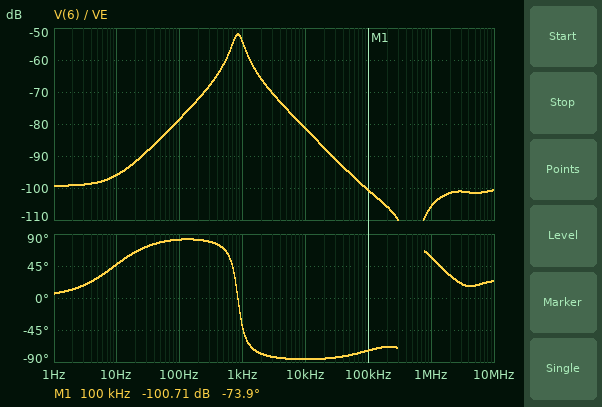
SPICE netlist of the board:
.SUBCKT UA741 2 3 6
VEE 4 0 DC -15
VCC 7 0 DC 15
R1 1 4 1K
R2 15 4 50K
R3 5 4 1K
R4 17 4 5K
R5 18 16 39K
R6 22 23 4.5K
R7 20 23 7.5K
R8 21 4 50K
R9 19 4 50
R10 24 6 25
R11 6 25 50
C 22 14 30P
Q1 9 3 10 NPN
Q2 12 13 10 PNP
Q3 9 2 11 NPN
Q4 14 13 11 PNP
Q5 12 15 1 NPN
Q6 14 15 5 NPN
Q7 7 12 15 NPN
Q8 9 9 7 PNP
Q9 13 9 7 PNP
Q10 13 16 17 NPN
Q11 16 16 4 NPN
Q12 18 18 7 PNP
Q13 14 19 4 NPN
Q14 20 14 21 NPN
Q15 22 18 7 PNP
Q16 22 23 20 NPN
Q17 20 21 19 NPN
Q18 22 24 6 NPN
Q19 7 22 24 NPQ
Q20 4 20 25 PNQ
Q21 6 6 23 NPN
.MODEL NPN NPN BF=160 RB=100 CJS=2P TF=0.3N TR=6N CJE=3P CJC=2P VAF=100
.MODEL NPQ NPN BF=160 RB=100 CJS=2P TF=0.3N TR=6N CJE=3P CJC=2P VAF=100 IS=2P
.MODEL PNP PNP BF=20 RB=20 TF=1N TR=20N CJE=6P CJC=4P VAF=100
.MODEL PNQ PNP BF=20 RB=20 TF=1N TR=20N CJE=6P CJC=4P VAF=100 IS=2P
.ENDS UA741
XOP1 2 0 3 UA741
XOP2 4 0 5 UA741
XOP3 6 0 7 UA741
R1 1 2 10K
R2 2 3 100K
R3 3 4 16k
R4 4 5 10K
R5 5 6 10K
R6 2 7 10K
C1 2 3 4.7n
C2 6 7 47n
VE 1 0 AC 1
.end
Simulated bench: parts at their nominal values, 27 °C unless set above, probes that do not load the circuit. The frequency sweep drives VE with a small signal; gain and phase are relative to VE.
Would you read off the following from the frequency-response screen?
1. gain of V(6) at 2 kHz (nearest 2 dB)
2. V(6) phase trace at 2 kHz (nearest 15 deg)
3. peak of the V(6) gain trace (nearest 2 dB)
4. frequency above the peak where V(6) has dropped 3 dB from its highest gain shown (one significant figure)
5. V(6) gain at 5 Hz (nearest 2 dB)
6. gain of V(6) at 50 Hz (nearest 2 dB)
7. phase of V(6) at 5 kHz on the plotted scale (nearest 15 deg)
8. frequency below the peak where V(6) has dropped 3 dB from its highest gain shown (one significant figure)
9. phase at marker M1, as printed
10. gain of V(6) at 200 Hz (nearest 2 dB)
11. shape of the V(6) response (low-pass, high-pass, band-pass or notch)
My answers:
-66 dB
-75 deg
-52 dB
1 kHz
-98 dB
-84 dB
-90 deg
700 Hz
-73.9 deg
-72 dB
band-pass
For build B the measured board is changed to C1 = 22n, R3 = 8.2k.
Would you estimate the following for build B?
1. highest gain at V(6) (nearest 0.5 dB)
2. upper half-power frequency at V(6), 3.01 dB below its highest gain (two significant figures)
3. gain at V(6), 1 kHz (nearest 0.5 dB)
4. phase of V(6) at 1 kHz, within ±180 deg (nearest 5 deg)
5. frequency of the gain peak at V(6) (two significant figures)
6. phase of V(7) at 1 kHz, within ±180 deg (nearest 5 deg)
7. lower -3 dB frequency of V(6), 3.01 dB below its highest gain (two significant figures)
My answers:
-46.0 dB
580 Hz
-66.0 dB
-85 deg
550 Hz
5 deg
510 Hz
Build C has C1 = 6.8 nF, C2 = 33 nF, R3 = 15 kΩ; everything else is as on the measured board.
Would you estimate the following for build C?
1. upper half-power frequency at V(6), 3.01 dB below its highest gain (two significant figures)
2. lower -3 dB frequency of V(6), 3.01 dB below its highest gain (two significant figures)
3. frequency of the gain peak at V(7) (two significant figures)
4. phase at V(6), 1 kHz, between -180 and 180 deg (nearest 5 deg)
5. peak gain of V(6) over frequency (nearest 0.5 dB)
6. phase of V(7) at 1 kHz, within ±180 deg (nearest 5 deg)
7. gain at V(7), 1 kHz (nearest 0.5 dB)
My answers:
990 Hz
760 Hz
850 Hz
-50 deg
-48.5 dB
40 deg
7.0 dB
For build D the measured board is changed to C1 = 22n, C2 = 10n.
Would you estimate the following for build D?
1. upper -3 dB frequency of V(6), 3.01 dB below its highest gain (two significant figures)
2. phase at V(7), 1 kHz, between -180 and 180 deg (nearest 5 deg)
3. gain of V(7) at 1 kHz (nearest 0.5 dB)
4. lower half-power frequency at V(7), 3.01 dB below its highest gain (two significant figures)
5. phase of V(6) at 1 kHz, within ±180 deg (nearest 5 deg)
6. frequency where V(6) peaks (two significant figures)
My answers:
880 Hz
15 deg
8.0 dB
810 Hz
-75 deg
850 Hz
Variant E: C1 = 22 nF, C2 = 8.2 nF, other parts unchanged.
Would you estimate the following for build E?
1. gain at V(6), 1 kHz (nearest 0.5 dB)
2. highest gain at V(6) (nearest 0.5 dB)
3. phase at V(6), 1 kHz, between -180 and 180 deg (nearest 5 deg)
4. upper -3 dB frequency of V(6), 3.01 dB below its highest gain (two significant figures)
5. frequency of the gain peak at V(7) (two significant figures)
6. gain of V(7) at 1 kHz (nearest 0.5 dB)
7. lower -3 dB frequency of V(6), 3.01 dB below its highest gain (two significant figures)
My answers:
-43.0 dB
-36.5 dB
-60 deg
970 Hz
930 Hz
15.5 dB
900 Hz
